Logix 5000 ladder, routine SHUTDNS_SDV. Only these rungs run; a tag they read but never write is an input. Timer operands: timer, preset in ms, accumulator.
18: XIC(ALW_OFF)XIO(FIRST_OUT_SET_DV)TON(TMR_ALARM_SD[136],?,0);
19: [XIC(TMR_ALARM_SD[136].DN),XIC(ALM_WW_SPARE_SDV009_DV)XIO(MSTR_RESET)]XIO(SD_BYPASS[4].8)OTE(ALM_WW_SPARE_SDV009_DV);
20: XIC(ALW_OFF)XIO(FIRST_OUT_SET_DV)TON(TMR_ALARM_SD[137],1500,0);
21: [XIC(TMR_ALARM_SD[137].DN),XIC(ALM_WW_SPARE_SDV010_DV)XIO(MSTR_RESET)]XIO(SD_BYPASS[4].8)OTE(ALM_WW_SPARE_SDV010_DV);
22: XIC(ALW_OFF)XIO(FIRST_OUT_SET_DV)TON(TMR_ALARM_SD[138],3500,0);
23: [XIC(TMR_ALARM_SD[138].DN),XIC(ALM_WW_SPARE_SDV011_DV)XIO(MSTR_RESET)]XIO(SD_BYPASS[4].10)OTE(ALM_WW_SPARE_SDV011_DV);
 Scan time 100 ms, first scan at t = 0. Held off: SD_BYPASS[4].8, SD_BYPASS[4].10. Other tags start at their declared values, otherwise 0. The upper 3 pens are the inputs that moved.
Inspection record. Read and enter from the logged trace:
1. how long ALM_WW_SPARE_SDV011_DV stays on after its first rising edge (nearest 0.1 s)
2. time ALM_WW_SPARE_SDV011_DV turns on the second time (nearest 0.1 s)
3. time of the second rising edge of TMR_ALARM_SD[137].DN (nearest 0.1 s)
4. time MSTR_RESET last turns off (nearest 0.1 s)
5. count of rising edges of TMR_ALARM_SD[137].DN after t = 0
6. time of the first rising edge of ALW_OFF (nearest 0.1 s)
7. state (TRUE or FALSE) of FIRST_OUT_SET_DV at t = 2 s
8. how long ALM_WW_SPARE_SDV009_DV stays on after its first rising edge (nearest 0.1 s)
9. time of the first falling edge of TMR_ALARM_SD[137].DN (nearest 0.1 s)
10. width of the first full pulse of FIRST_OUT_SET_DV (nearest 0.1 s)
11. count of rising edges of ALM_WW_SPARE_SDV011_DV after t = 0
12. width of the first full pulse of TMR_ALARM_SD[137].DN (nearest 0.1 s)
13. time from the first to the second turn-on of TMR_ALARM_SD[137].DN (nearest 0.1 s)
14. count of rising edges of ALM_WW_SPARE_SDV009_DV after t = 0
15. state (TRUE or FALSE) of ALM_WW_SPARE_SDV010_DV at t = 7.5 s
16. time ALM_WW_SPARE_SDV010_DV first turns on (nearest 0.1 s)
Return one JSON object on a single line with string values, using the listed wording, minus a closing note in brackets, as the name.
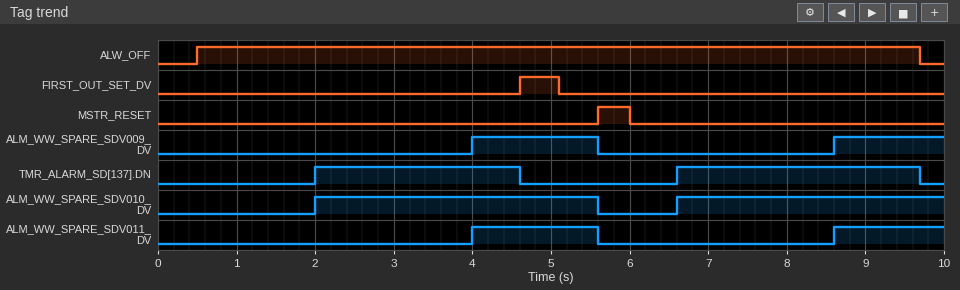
{"how long ALM_WW_SPARE_SDV011_DV stays on after its first rising edge": "1.6 s", "time ALM_WW_SPARE_SDV011_DV turns on the second time": "8.6 s", "time of the second rising edge of TMR_ALARM_SD[137].DN": "6.6 s", "time MSTR_RESET last turns off": "6.0 s", "count of rising edges of TMR_ALARM_SD[137].DN after t = 0": "2", "time of the first rising edge of ALW_OFF": "0.5 s", "state (TRUE or FALSE) of FIRST_OUT_SET_DV at t = 2 s": "FALSE", "how long ALM_WW_SPARE_SDV009_DV stays on after its first rising edge": "1.6 s", "time of the first falling edge of TMR_ALARM_SD[137].DN": "4.6 s", "width of the first full pulse of FIRST_OUT_SET_DV": "0.5 s", "count of rising edges of ALM_WW_SPARE_SDV011_DV after t = 0": "2", "width of the first full pulse of TMR_ALARM_SD[137].DN": "2.6 s", "time from the first to the second turn-on of TMR_ALARM_SD[137].DN": "4.6 s", "count of rising edges of ALM_WW_SPARE_SDV009_DV after t = 0": "2", "state (TRUE or FALSE) of ALM_WW_SPARE_SDV010_DV at t = 7.5 s": "TRUE", "time ALM_WW_SPARE_SDV010_DV first turns on": "2.0 s"}
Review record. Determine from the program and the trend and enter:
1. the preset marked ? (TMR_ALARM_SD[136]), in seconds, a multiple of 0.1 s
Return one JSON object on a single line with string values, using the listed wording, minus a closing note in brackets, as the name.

{"the preset marked ? (TMR_ALARM_SD[136]), in seconds, a multiple of 0.1 s": "3.5 s"}
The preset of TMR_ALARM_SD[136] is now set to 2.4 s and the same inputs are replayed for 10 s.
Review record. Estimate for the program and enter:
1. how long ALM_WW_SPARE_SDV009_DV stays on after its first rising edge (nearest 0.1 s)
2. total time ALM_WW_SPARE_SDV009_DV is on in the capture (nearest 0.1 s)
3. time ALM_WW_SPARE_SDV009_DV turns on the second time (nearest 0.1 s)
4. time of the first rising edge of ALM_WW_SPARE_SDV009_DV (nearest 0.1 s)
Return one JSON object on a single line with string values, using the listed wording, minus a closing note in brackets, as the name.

{"how long ALM_WW_SPARE_SDV009_DV stays on after its first rising edge": "2.7 s", "total time ALM_WW_SPARE_SDV009_DV is on in the capture": "5.2 s", "time ALM_WW_SPARE_SDV009_DV turns on the second time": "7.5 s", "time of the first rising edge of ALM_WW_SPARE_SDV009_DV": "2.9 s"}
